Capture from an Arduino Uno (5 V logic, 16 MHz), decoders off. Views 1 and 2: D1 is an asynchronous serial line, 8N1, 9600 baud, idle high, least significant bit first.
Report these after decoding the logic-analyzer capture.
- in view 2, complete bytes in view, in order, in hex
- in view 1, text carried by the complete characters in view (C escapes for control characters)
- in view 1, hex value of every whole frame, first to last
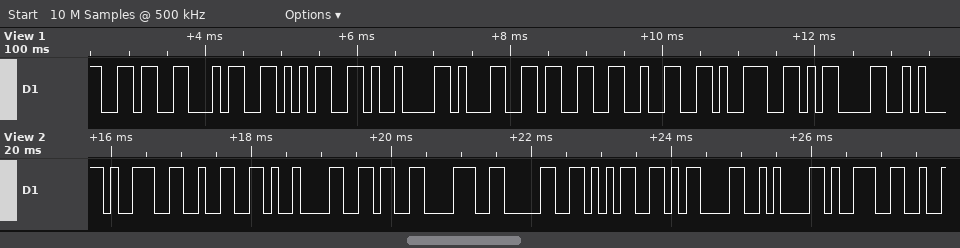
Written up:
39 32 09 36 38 30 35 0D 0A 39
"645\t1329\r"
0x36 0x34 0x35 0x09 0x31 0x33 0x32 0x39 0x0D
